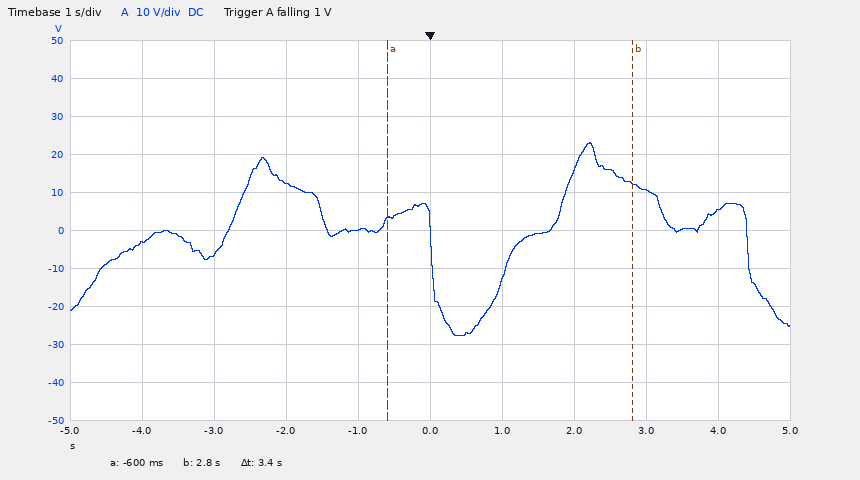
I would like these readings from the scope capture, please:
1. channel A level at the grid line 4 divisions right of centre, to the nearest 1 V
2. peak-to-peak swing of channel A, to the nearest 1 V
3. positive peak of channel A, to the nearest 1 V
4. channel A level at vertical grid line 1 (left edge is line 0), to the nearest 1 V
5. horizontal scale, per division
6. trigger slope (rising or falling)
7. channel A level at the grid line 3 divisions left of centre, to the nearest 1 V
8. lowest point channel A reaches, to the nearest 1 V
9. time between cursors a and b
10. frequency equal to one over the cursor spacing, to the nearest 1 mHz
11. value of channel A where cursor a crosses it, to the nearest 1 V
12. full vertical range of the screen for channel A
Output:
5 V
51 V
23 V
-3 V
1 s
falling
-6 V
-28 V
3.4 s
294 mHz
3 V
100 V
